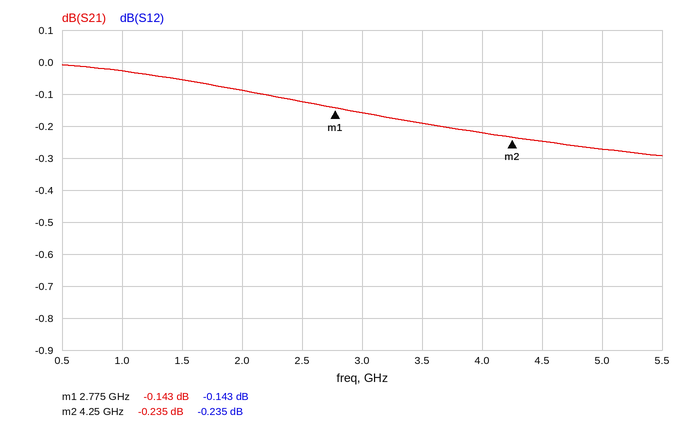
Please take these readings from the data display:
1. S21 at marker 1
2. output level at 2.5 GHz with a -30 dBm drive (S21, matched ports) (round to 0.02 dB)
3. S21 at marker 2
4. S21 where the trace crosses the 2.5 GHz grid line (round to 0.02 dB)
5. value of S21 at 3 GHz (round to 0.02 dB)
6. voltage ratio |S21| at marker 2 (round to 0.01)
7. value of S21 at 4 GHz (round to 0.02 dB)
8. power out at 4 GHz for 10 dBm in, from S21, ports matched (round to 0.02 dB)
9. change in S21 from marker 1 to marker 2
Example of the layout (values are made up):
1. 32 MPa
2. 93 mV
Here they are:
1. -0.143 dB
2. -30.12 dBm
3. -0.235 dB
4. -0.12 dB
5. -0.16 dB
6. 0.97
7. -0.22 dB
8. 9.78 dBm
9. -0.092 dB
